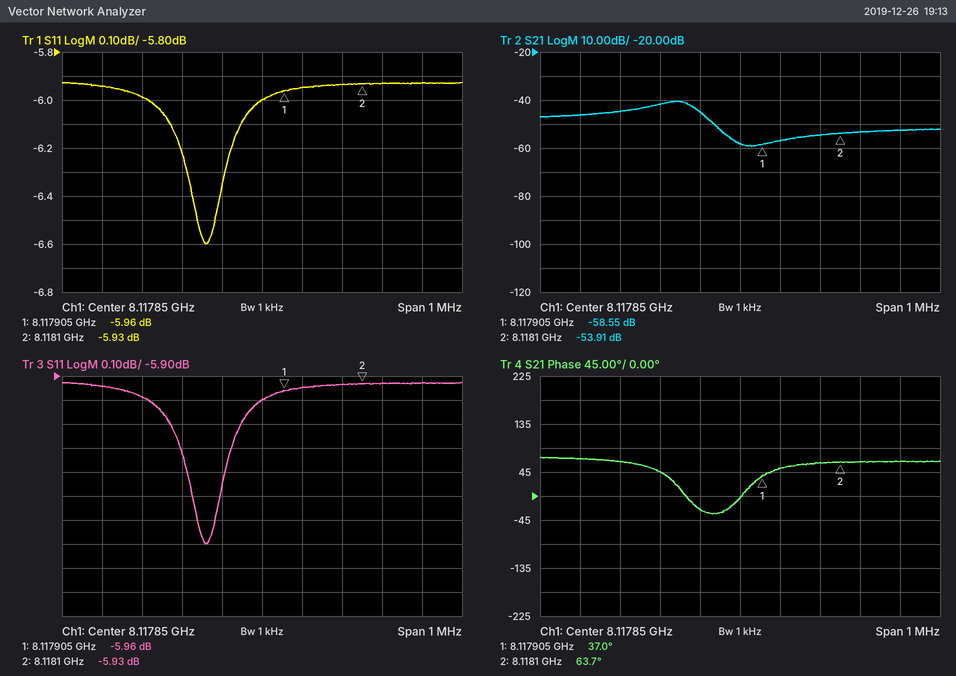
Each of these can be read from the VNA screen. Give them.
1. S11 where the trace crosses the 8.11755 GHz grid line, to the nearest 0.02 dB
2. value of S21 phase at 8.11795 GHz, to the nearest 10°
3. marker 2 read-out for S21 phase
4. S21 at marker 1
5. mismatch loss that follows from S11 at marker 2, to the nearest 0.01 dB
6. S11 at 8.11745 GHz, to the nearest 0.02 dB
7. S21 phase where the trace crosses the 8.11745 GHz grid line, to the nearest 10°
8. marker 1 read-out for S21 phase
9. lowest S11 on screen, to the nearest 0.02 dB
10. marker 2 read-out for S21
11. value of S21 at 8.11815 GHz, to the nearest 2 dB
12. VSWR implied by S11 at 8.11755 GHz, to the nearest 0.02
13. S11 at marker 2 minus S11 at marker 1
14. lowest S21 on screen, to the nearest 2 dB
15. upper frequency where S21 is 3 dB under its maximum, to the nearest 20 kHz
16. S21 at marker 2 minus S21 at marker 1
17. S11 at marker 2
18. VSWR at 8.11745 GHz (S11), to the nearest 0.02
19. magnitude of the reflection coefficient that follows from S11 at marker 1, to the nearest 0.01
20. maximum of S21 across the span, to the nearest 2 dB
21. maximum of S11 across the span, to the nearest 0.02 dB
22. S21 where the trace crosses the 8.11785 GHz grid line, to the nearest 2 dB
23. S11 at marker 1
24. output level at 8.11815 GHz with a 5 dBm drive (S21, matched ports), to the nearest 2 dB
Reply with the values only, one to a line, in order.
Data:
-5.98 dB
50°
63.7°
-58.55 dB
1.28 dB
-5.94 dB
70°
37.0°
-6.60 dB
-53.91 dB
-54 dB
3.02
0.03 dB
-60 dB
8.11774 GHz
4.64 dB
-5.93 dB
3.04
0.50
-40 dB
-5.92 dB
-58 dB
-5.96 dB
-48 dBm
